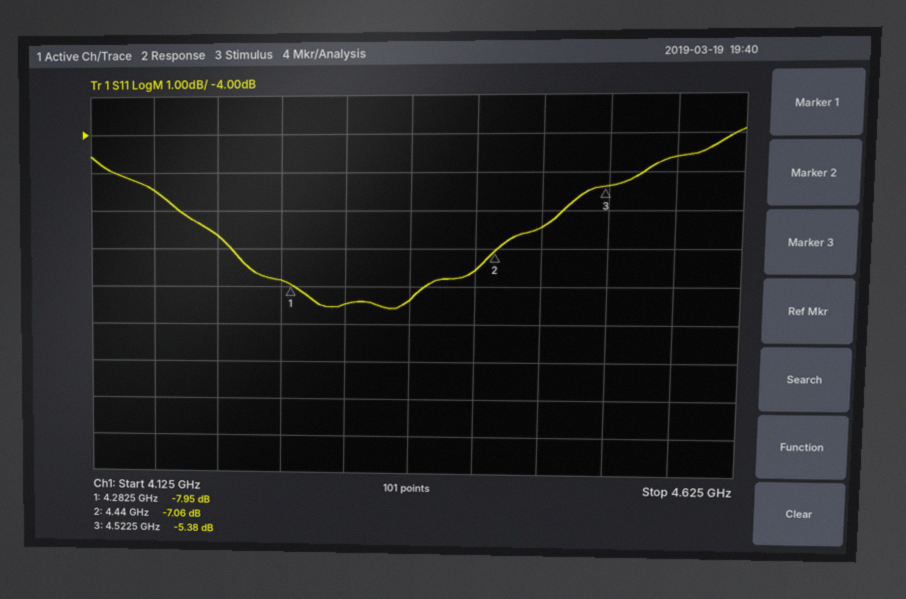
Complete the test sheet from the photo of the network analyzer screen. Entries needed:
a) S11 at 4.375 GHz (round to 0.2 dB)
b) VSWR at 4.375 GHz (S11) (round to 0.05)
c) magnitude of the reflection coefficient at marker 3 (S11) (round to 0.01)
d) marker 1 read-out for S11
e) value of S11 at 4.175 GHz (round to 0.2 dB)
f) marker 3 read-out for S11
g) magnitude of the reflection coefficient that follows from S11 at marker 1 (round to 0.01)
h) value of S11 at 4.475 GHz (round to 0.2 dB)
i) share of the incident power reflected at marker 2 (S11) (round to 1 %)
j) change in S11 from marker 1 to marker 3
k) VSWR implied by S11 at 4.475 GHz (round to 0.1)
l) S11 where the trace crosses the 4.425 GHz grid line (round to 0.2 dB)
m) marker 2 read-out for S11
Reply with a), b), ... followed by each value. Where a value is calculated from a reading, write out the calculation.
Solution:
a) -8.4 dB
b) |Γ| = 10^(-8.4/20) = 0.3802; VSWR = (1 + 0.3802)/(1 − 0.3802) ≈ 2.23, so 2.25 to the nearest 0.05
c) 10^(-5.38/20) ≈ 0.54
d) -7.95 dB
e) -5.4 dB
f) -5.38 dB
g) 10^(-7.95/20) ≈ 0.40
h) -6.4 dB
i) 10^(-7.06/10) ≈ 20 %
j) -5.38 − (-7.95) = 2.57 dB
k) |Γ| = 10^(-6.4/20) = 0.4786; VSWR = (1 + 0.4786)/(1 − 0.4786) ≈ 2.8
l) -7.6 dB
m) -7.06 dB
